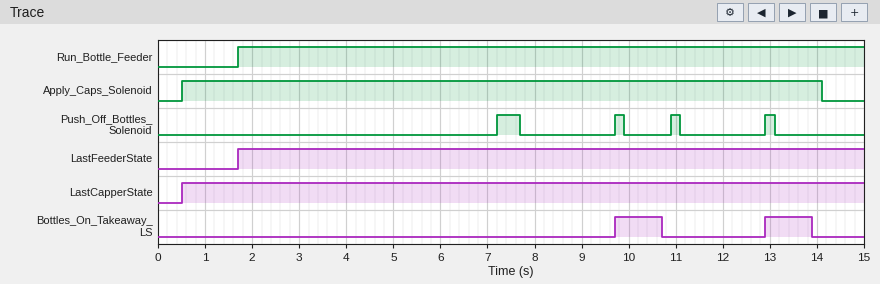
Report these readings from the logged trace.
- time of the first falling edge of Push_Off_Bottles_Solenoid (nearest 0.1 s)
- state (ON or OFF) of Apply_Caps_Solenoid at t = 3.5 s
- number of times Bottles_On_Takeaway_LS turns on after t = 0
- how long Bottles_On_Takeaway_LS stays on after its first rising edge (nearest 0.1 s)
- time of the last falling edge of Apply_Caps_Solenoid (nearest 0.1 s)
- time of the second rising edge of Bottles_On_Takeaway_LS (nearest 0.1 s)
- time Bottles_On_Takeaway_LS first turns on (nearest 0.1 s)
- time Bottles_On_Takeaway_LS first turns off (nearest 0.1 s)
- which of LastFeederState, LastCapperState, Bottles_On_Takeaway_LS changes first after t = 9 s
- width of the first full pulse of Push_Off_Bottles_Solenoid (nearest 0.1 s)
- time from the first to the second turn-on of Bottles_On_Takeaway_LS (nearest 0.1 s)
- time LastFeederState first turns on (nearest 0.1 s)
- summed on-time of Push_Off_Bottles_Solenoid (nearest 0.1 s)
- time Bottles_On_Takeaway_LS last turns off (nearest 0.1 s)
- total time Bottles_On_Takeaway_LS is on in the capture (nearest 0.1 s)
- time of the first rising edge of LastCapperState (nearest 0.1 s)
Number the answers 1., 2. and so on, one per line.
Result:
1. 7.7 s
2. ON
3. 2
4. 1.0 s
5. 14.1 s
6. 12.9 s
7. 9.7 s
8. 10.7 s
9. Bottles_On_Takeaway_LS
10. 0.5 s
11. 3.2 s
12. 1.7 s
13. 1.1 s
14. 13.9 s
15. 2.0 s
16. 0.5 s
